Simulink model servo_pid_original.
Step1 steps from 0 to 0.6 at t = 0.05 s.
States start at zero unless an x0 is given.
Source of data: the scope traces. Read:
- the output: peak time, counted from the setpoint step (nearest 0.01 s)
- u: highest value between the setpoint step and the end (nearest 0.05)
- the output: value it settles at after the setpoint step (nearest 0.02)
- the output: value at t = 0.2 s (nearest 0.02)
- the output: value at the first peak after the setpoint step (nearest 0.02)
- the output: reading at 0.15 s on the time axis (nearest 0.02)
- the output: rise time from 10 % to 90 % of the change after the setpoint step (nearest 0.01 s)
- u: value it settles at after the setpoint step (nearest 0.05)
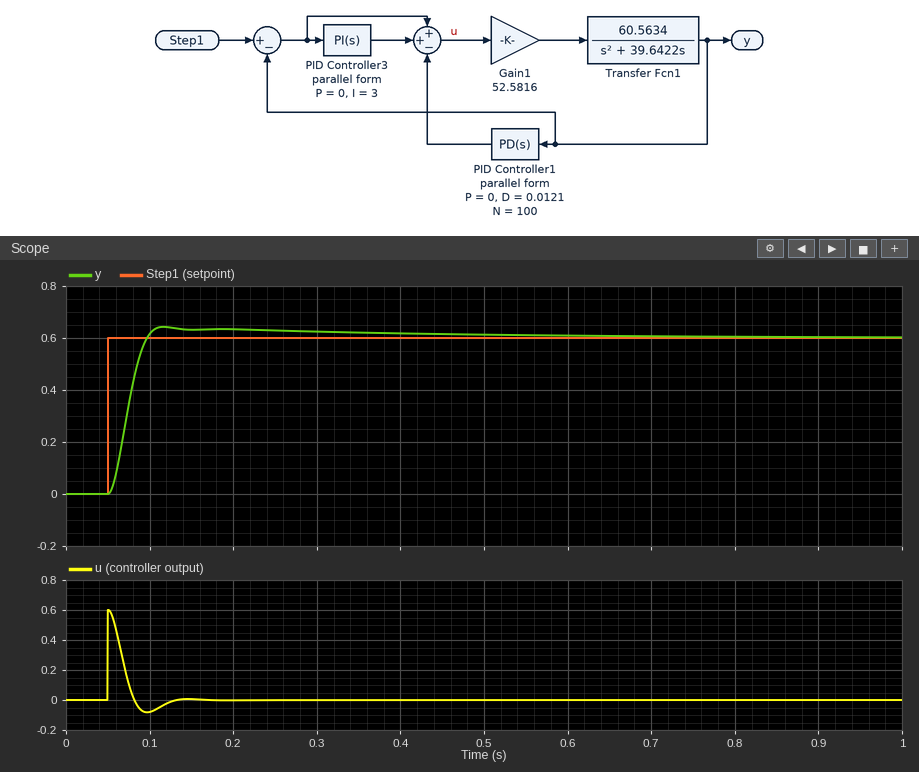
0.07 s
0.60
0.60
0.64
0.64
0.64
0.03 s
0.00
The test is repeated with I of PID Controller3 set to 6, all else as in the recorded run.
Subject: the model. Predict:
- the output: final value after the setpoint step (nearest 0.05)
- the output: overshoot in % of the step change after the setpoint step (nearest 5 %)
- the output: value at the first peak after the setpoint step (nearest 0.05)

0.60
15 %
0.70
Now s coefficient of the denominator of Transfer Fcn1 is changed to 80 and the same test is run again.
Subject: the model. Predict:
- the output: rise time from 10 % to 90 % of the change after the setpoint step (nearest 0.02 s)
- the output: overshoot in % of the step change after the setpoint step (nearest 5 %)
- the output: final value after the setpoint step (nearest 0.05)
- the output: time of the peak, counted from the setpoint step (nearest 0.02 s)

0.06 s
10 %
0.60
0.18 s
